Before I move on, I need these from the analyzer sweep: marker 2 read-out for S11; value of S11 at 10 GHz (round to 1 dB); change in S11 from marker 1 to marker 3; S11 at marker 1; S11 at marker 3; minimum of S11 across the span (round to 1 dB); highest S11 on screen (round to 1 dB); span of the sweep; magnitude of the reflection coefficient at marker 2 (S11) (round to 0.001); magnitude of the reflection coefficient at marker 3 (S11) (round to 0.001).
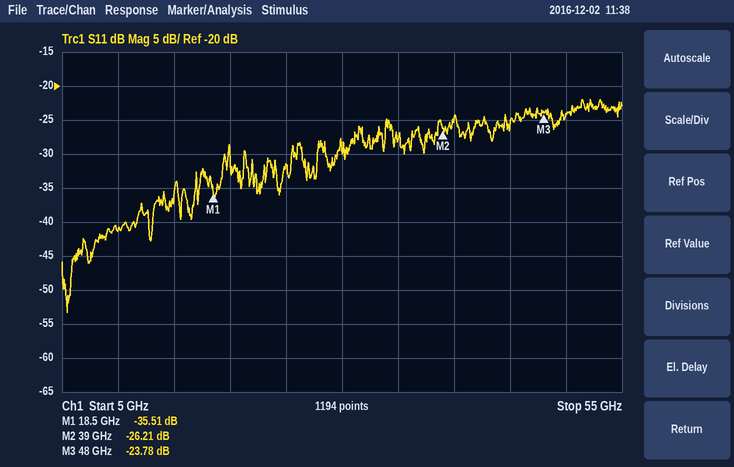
-26.21 dB
-41 dB
11.73 dB
-35.51 dB
-23.78 dB
-53 dB
-22 dB
50 GHz
0.049
0.065
